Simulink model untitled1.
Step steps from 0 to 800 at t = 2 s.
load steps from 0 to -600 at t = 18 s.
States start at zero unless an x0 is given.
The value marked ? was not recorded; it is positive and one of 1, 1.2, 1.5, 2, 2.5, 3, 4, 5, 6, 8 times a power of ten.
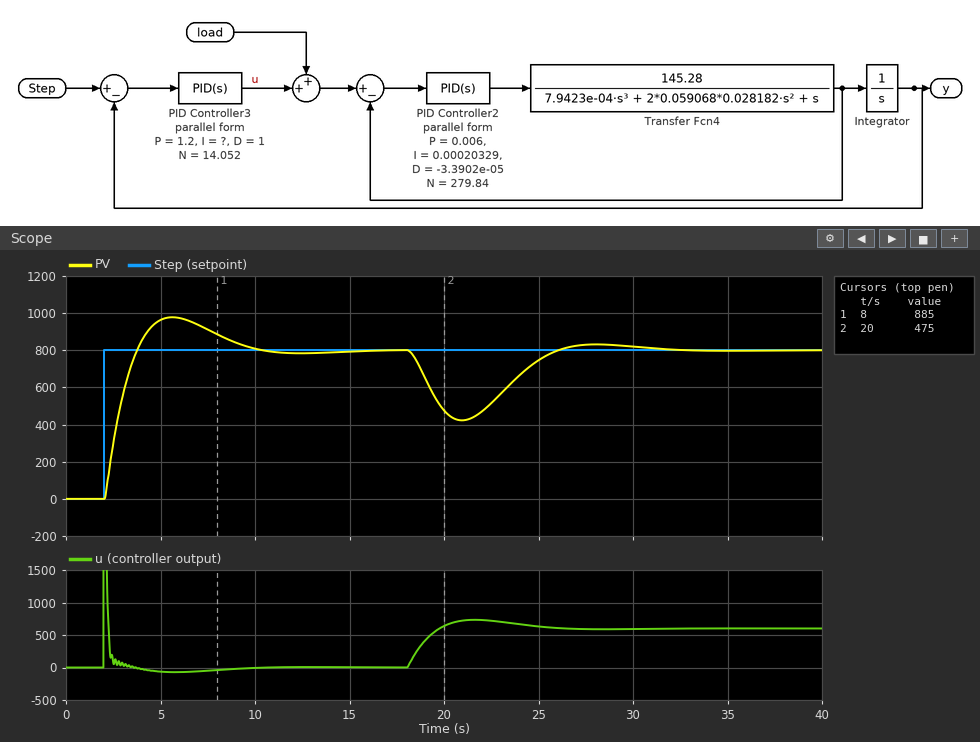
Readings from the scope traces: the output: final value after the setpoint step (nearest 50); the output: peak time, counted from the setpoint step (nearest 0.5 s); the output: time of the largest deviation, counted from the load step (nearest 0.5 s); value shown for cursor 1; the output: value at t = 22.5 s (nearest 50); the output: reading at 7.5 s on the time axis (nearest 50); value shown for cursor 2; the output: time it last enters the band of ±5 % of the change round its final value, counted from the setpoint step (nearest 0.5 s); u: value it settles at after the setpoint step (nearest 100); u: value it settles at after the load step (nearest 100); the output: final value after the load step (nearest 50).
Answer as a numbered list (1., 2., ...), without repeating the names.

1. 800
2. 3.5 s
3. 3.0 s
4. 885
5. 500
6. 900
7. 475
8. 7.0 s
9. 0
10. 600
11. 800
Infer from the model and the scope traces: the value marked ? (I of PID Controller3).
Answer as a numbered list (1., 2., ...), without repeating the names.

1. 0.4
